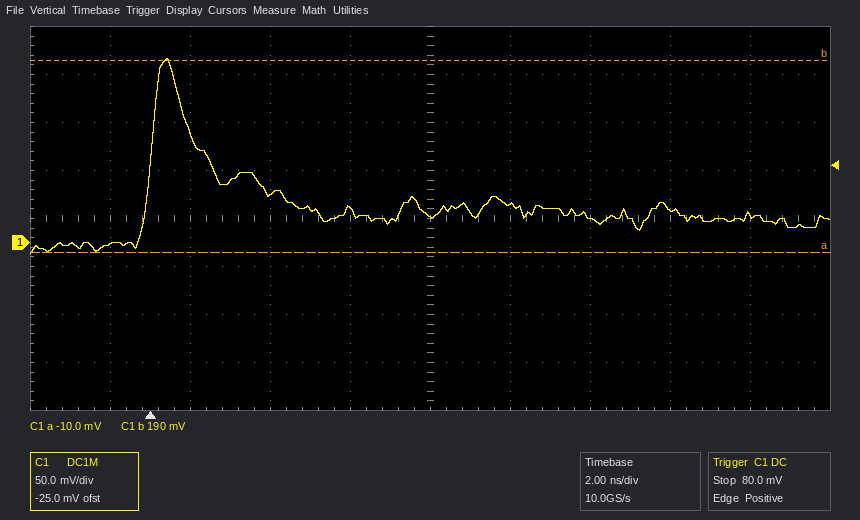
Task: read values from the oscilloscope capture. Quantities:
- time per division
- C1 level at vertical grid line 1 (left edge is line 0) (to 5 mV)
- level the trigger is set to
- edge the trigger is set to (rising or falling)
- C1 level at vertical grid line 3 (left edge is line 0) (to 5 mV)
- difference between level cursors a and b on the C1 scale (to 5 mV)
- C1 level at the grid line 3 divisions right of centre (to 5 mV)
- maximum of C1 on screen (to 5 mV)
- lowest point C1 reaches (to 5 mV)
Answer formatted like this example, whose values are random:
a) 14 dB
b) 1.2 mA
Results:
a) 2 ns
b) 0 mV
c) 80.0 mV
d) rising
e) 50 mV
f) 200 mV
g) 35 mV
h) 190 mV
i) -10 mV
